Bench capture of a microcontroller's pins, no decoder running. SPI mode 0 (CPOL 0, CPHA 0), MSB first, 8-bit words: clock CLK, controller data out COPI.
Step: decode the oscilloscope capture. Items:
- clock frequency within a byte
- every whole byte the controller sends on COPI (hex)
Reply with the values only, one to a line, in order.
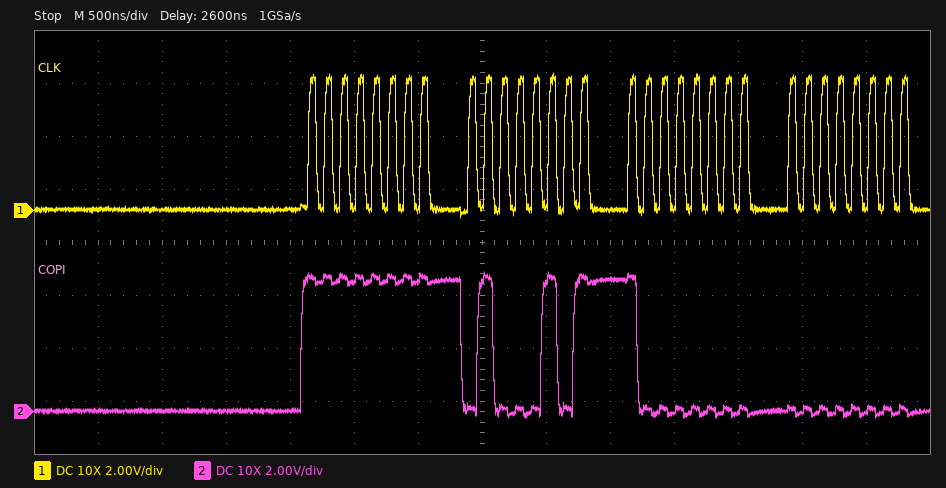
8 MHz
FF 45 80 00
